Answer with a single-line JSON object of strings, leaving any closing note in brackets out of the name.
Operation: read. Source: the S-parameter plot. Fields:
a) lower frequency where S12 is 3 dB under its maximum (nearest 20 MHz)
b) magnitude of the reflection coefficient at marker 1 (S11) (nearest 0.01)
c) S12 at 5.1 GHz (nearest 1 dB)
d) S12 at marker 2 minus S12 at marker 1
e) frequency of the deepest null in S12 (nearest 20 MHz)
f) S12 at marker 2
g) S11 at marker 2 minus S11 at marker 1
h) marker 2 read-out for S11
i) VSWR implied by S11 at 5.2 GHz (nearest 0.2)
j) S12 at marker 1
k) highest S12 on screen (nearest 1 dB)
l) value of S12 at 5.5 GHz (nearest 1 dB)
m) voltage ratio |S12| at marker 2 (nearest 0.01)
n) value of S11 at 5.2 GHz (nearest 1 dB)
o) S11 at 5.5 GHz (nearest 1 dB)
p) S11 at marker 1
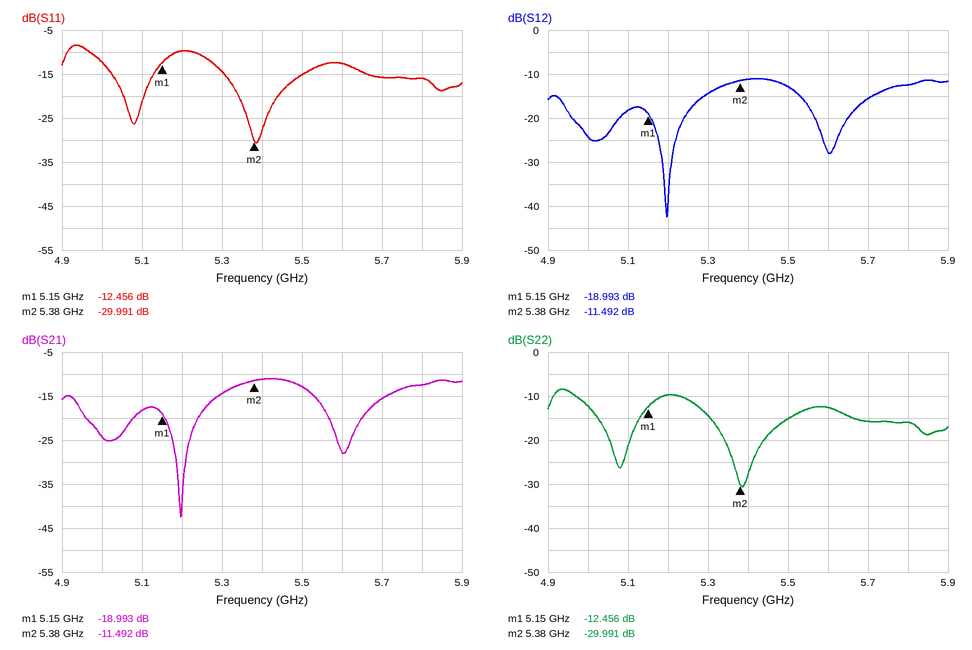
{"lower frequency where S12 is 3 dB under its maximum": "5.30 GHz", "magnitude of the reflection coefficient at marker 1 (S11)": "0.24", "S12 at 5.1 GHz": "-18 dB", "S12 at marker 2 minus S12 at marker 1": "7.501 dB", "frequency of the deepest null in S12": "5.20 GHz", "S12 at marker 2": "-11.492 dB", "S11 at marker 2 minus S11 at marker 1": "-17.535 dB", "marker 2 read-out for S11": "-29.991 dB", "VSWR implied by S11 at 5.2 GHz": "2.0", "S12 at marker 1": "-18.993 dB", "highest S12 on screen": "-11 dB", "value of S12 at 5.5 GHz": "-13 dB", "voltage ratio |S12| at marker 2": "0.27", "value of S11 at 5.2 GHz": "-10 dB", "S11 at 5.5 GHz": "-15 dB", "S11 at marker 1": "-12.456 dB"}
